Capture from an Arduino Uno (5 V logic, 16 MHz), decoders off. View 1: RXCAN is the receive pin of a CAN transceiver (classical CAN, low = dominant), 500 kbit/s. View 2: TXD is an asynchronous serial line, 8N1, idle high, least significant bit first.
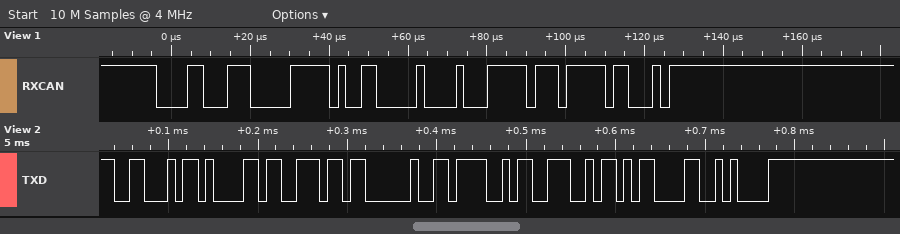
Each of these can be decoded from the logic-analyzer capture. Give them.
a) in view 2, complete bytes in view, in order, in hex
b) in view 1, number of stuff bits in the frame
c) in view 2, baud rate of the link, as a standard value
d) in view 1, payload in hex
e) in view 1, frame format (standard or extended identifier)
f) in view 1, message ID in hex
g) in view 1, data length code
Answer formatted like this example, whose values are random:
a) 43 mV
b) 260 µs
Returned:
a) 46 61 6E 20 4F 4E 0D 0A
b) 5
c) 115200 baud
d) E6 00 8F
e) standard
f) 0x0C7
g) 3
